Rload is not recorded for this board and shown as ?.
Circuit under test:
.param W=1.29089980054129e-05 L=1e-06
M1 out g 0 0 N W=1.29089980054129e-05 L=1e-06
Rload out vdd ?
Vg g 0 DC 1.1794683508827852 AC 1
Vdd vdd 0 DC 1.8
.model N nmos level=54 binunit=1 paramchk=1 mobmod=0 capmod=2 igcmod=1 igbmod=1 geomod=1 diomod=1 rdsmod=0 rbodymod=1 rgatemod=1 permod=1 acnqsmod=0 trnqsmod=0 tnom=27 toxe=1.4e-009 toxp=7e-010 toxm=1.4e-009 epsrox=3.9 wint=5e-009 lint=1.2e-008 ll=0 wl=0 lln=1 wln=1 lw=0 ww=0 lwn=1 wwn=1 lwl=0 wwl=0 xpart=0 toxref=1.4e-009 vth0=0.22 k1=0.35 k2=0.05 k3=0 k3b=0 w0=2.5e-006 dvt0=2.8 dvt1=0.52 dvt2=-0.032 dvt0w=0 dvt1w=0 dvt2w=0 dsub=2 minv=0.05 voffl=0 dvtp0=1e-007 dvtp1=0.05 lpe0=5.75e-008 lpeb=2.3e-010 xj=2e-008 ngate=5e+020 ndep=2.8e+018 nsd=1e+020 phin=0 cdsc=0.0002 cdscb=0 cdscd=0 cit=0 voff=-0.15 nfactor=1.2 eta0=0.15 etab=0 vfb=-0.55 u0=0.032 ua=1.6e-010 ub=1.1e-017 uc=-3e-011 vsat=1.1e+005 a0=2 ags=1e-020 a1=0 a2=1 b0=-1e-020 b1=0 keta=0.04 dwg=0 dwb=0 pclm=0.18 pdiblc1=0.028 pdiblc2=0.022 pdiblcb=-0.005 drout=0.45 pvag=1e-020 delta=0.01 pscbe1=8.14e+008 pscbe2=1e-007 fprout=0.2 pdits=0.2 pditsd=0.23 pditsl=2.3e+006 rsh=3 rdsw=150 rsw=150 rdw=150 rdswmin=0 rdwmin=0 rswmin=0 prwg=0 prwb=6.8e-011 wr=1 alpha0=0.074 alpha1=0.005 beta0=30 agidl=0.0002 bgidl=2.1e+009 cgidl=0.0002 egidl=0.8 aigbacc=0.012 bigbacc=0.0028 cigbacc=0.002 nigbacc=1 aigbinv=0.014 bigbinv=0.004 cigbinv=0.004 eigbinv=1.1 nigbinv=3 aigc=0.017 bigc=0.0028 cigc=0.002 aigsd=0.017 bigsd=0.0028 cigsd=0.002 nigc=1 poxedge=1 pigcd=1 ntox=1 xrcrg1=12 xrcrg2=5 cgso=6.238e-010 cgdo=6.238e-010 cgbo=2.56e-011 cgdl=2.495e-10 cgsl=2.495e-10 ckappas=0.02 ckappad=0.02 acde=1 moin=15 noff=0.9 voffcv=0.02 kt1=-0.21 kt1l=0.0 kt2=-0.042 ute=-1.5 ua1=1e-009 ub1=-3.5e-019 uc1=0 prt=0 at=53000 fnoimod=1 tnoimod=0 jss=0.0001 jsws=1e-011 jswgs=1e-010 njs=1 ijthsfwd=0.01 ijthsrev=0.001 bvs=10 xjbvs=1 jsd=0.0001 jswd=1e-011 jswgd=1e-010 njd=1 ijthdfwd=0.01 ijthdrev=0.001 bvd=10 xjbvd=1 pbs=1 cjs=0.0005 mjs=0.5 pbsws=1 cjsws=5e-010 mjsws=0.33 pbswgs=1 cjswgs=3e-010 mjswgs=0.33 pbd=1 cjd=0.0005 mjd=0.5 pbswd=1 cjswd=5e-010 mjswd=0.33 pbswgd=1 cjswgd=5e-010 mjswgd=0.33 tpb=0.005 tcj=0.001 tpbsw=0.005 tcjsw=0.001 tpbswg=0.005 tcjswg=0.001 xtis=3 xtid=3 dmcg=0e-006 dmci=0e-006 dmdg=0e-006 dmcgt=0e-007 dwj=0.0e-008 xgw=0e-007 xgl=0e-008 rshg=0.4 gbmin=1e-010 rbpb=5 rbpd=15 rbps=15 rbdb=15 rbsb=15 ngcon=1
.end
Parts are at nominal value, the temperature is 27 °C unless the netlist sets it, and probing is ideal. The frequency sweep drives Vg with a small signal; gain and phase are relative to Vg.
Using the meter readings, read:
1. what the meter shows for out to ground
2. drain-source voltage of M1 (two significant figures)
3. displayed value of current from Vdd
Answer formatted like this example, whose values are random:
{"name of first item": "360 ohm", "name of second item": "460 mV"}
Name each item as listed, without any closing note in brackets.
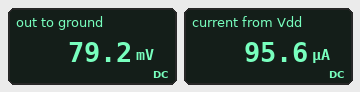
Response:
{"what the meter shows for out to ground": "79.2 mV", "drain-source voltage of M1": "79 mV", "displayed value of current from Vdd": "95.6 µA"}
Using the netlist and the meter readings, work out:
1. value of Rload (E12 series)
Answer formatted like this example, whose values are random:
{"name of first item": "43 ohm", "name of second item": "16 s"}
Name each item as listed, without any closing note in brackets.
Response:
{"value of Rload": "18 kΩ"}
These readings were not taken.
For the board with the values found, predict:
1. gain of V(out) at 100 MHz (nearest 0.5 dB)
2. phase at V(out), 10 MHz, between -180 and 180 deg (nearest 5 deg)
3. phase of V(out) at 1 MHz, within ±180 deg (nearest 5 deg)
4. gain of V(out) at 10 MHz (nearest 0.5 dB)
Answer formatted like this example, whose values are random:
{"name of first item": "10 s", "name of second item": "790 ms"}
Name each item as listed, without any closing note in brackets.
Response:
{"gain of V(out) at 100 MHz": "-17.5 dB", "phase at V(out), 10 MHz, between -180 and 180 deg": "60 deg", "phase of V(out) at 1 MHz, within ±180 deg": "10 deg", "gain of V(out) at 10 MHz": "-36.0 dB"}
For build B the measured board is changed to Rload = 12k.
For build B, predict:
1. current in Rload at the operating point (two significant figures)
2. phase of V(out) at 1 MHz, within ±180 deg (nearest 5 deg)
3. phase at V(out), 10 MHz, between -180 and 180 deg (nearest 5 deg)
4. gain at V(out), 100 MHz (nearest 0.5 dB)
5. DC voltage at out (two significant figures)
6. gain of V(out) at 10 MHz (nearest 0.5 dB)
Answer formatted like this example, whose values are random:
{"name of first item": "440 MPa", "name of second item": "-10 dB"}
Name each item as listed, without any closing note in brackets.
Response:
{"current in Rload at the operating point": "140 µA", "phase of V(out) at 1 MHz, within ±180 deg": "15 deg", "phase at V(out), 10 MHz, between -180 and 180 deg": "70 deg", "gain at V(out), 100 MHz": "-17.0 dB", "DC voltage at out": "120 mV", "gain of V(out) at 10 MHz": "-36.5 dB"}
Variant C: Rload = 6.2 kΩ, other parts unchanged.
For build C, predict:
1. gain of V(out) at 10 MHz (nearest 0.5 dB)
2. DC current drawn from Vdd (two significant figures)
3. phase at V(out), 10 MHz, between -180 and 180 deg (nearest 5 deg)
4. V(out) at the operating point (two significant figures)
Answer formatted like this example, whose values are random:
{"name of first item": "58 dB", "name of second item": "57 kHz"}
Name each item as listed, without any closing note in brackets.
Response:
{"gain of V(out) at 10 MHz": "-31.0 dB", "DC current drawn from Vdd": "250 µA", "phase at V(out), 10 MHz, between -180 and 180 deg": "145 deg", "V(out) at the operating point": "240 mV"}
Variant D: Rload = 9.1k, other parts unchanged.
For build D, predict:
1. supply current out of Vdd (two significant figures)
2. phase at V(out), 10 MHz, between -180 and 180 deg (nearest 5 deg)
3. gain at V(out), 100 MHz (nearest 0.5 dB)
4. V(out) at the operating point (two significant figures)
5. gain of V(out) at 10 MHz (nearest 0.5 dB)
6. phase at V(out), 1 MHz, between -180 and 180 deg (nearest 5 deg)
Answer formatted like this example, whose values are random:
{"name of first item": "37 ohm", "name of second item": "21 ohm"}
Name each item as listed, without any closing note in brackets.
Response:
{"supply current out of Vdd": "180 µA", "phase at V(out), 10 MHz, between -180 and 180 deg": "90 deg", "gain at V(out), 100 MHz": "-17.0 dB", "V(out) at the operating point": "160 mV", "gain of V(out) at 10 MHz": "-36.5 dB", "phase at V(out), 1 MHz, between -180 and 180 deg": "100 deg"}
